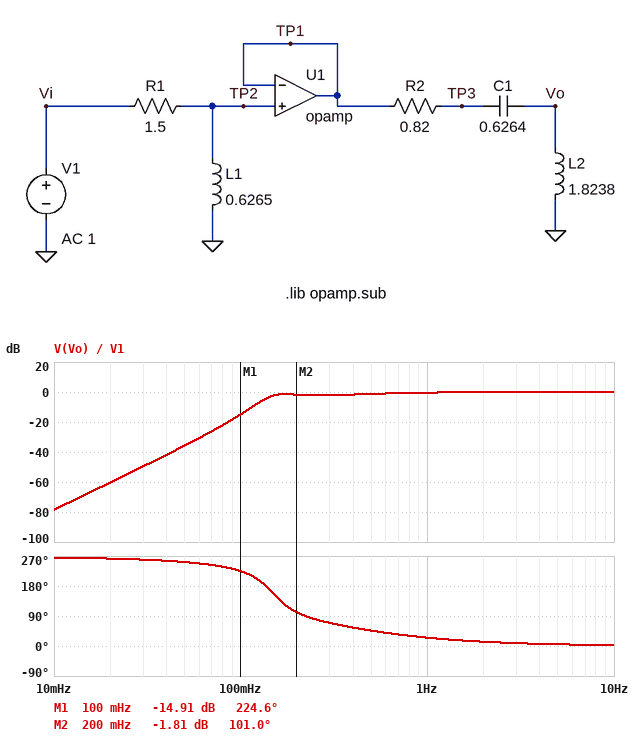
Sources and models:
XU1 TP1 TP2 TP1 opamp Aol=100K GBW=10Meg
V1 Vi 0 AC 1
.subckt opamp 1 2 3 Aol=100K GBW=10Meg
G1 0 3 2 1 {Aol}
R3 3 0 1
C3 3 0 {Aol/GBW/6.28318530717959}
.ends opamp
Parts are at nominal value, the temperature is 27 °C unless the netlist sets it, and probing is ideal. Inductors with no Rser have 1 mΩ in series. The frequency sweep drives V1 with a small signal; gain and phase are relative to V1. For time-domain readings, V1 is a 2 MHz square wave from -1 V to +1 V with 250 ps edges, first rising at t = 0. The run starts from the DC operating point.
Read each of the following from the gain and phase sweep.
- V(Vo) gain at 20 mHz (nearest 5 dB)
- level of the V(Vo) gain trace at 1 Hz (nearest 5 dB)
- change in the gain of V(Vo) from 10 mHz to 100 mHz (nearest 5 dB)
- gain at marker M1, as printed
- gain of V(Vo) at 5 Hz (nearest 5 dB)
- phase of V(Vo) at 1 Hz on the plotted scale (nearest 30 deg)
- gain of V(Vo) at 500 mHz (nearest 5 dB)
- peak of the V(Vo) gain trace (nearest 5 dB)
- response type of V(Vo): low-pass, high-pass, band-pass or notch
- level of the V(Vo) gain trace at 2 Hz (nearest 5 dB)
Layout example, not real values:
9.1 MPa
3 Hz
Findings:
-60 dB
0 dB
65 dB
-14.91 dB
0 dB
30 deg
0 dB
0 dB
high-pass
0 dB
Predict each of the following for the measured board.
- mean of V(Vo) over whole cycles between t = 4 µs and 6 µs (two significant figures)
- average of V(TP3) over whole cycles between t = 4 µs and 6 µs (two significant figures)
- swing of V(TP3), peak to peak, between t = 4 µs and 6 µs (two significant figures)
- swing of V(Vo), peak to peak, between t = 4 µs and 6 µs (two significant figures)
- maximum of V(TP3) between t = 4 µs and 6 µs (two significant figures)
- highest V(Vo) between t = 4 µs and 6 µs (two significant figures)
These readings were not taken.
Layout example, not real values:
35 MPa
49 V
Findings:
1.0 V
1.0 V
2.0 V
2.0 V
2.0 V
2.0 V
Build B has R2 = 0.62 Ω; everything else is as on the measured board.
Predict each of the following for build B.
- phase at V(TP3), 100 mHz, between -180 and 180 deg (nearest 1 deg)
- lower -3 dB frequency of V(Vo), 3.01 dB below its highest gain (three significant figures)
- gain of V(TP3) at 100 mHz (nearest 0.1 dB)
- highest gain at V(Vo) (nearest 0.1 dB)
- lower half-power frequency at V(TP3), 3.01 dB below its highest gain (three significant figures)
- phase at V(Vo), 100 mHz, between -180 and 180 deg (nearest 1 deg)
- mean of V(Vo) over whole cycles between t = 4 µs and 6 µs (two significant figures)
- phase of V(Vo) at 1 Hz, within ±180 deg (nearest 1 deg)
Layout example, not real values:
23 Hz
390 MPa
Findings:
51 deg
136 mHz
-12.7 dB
0.5 dB
391 mHz
-129 deg
1.0 V
24 deg
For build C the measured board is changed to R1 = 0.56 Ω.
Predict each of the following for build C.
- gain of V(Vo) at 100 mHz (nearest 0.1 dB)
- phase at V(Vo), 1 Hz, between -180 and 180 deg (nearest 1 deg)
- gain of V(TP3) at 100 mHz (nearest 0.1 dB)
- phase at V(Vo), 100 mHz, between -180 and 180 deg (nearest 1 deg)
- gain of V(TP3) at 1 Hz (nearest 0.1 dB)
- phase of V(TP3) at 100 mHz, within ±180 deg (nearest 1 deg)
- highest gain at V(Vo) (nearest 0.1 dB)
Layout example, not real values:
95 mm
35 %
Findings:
-7.8 dB
12 deg
-6.1 dB
-156 deg
-0.1 dB
24 deg
4.1 dB
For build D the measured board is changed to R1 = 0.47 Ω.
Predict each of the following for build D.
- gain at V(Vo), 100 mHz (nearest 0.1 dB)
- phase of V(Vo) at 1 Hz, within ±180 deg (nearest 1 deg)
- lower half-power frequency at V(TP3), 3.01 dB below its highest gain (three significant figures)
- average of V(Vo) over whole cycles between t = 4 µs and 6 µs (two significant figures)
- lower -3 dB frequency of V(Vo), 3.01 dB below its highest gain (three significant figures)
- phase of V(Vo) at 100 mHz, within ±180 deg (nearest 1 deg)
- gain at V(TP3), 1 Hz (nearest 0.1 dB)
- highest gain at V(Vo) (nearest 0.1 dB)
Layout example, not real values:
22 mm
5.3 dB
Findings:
-6.9 dB
11 deg
208 mHz
1.0 V
132 mHz
-161 deg
-0.1 dB
4.7 dB
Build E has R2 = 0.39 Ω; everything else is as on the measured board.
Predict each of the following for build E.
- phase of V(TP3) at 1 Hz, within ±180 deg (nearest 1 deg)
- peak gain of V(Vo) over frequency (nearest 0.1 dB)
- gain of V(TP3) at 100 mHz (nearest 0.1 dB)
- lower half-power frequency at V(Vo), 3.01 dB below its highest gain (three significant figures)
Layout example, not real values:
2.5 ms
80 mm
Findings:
23 deg
4.2 dB
-12.2 dB
138 mHz
